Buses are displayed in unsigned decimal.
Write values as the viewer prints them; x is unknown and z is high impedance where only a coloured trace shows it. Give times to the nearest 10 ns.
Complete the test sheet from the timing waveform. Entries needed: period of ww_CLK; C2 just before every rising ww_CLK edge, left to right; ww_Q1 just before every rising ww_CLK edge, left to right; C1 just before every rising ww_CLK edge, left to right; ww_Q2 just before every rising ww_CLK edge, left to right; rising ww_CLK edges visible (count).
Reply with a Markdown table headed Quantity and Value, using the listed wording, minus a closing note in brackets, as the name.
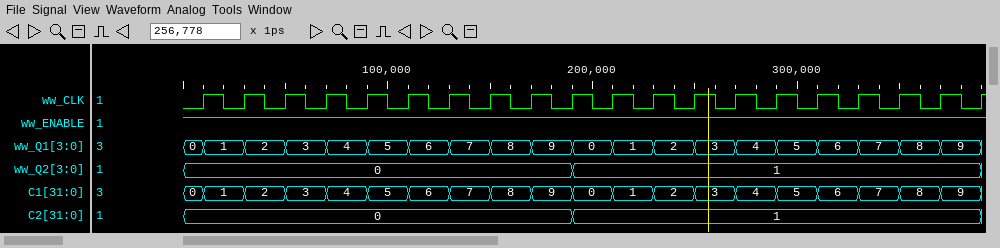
| Quantity | Value |
|---|---|
| period of ww_CLK | 20 ns |
| C2 just before every rising ww_CLK edge, left to right | 0, 0, 0, 0, 0, 0, 0, 0, 0, 0, 1, 1, 1, 1, 1, 1, 1, 1, 1, 1 |
| ww_Q1 just before every rising ww_CLK edge, left to right | 0, 1, 2, 3, 4, 5, 6, 7, 8, 9, 0, 1, 2, 3, 4, 5, 6, 7, 8, 9 |
| C1 just before every rising ww_CLK edge, left to right | 0, 1, 2, 3, 4, 5, 6, 7, 8, 9, 0, 1, 2, 3, 4, 5, 6, 7, 8, 9 |
| ww_Q2 just before every rising ww_CLK edge, left to right | 0, 0, 0, 0, 0, 0, 0, 0, 0, 0, 1, 1, 1, 1, 1, 1, 1, 1, 1, 1 |
| rising ww_CLK edges visible | 20 |
